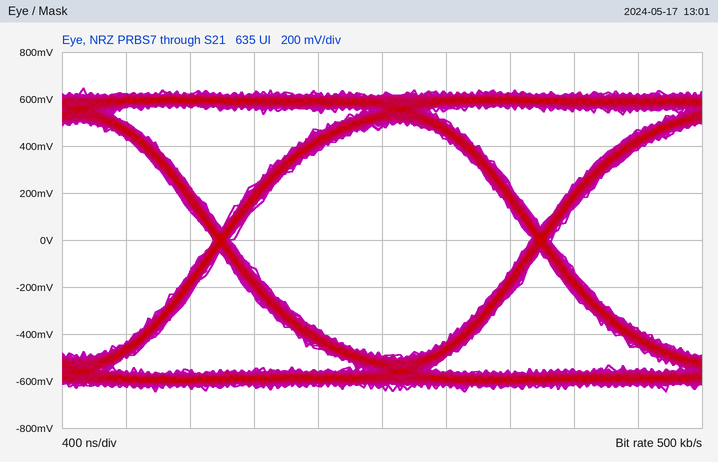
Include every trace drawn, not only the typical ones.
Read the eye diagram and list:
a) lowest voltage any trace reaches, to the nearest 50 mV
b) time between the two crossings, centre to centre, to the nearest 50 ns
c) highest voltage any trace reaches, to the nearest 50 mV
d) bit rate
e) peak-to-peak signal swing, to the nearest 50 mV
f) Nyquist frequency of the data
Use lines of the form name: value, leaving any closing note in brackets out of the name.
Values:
lowest voltage any trace reaches, to the nearest 50 mV: -650 mV
time between the two crossings, centre to centre, to the nearest 50 ns: 2.00 µs
highest voltage any trace reaches, to the nearest 50 mV: 650 mV
bit rate: 500 kb/s
peak-to-peak signal swing, to the nearest 50 mV: 1.30 V
Nyquist frequency of the data: 250 kHz
